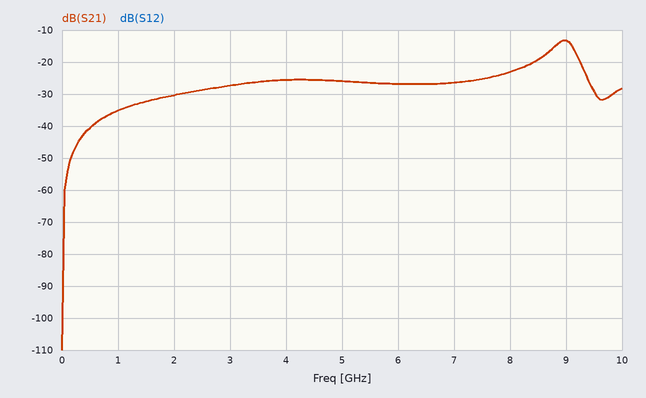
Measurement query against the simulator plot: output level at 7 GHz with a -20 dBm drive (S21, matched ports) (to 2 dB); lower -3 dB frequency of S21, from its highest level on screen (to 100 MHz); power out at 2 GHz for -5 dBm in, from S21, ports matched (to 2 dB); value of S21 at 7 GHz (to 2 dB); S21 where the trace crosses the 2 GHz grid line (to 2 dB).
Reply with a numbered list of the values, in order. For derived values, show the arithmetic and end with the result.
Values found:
1. -20 dBm + (-26 dB) = -46 dBm
2. 8.7 GHz
3. -5 dBm + (-30 dB) = -36 dBm
4. -26 dB
5. -30 dB
